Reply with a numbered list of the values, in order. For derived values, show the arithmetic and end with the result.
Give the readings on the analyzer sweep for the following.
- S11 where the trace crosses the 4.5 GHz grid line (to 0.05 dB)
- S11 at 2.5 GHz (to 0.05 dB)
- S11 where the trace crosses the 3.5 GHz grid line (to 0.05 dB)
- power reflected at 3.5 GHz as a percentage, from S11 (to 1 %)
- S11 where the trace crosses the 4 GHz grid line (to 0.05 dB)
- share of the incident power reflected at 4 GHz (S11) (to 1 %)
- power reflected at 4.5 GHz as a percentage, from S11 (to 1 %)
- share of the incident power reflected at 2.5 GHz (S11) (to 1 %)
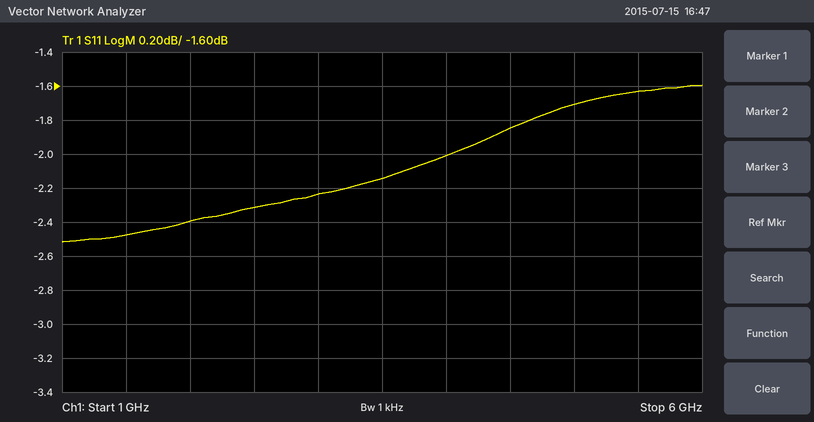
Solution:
1. -1.85 dB
2. -2.30 dB
3. -2.15 dB
4. 10^(-2.15/10) ≈ 61 %
5. -2.00 dB
6. 10^(-2/10) ≈ 63 %
7. 10^(-1.85/10) ≈ 65 %
8. 10^(-2.3/10) ≈ 59 %
